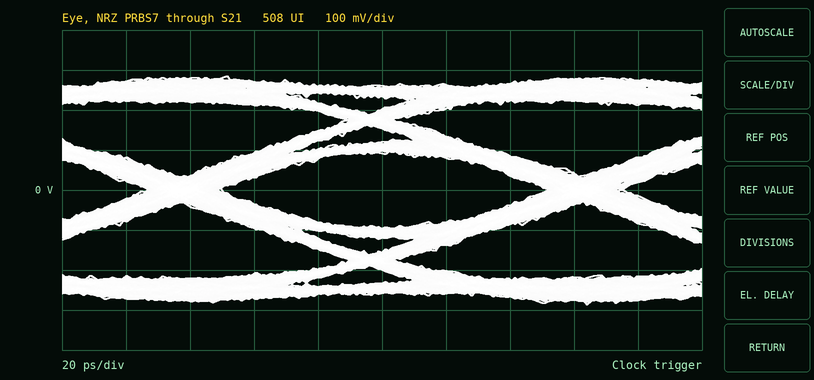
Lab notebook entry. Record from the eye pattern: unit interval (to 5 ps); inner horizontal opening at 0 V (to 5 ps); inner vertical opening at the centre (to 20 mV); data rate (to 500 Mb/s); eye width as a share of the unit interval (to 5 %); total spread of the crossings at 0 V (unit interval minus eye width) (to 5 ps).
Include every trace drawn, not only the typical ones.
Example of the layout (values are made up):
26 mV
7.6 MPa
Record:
125 ps
100 ps
180 mV
8.0 Gb/s
80 %
25 ps
